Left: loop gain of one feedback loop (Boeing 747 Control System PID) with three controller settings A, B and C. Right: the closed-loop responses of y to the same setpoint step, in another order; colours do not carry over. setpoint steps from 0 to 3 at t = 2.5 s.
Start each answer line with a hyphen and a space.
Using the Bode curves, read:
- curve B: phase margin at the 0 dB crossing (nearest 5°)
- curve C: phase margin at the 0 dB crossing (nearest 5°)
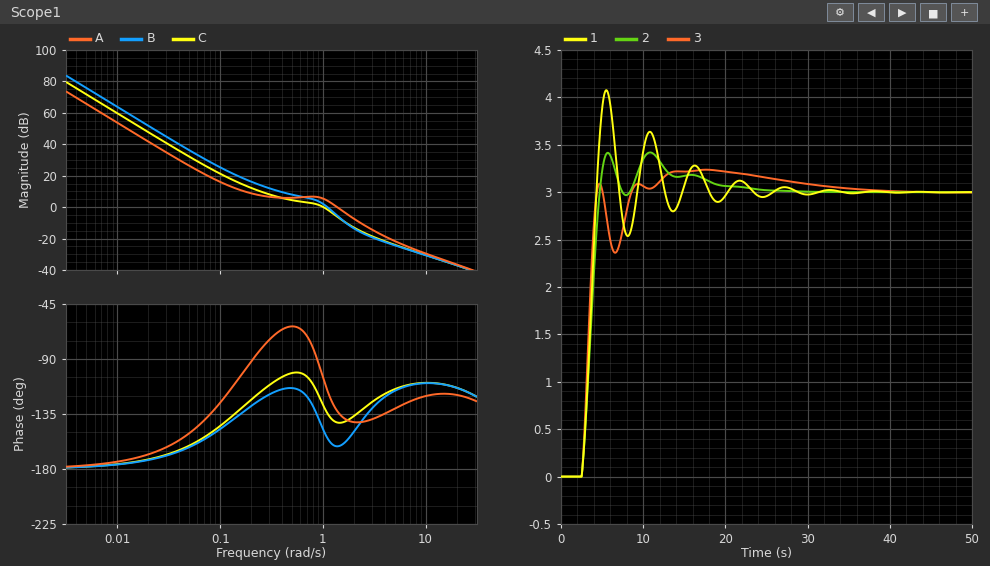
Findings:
- 25°
- 50°
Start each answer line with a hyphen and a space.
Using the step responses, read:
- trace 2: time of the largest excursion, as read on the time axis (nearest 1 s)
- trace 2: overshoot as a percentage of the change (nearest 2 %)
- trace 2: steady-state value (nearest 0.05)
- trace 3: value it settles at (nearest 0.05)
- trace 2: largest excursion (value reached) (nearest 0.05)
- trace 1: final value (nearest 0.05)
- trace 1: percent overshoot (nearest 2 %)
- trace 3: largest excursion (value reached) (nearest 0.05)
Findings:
- 11 s
- 14 %
- 3.00
- 3.00
- 3.40
- 3.00
- 36 %
- 3.25
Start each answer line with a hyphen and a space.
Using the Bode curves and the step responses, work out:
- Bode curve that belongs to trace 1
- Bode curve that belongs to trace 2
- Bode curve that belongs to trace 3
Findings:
- B
- C
- A
